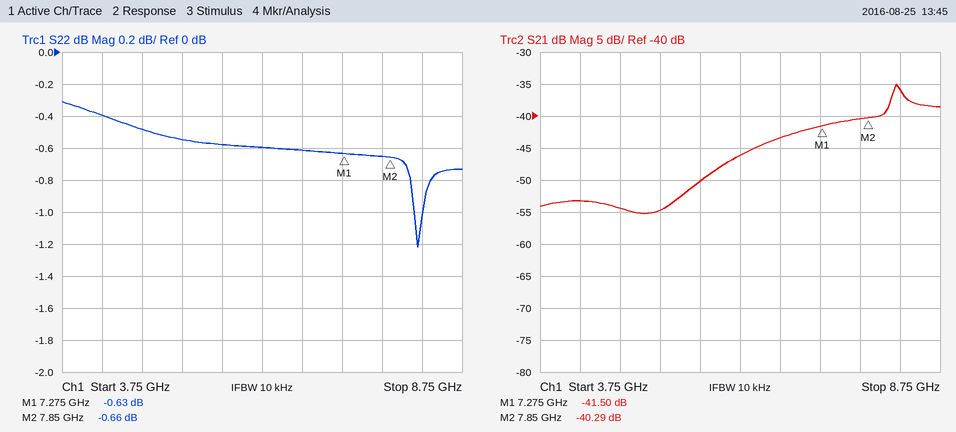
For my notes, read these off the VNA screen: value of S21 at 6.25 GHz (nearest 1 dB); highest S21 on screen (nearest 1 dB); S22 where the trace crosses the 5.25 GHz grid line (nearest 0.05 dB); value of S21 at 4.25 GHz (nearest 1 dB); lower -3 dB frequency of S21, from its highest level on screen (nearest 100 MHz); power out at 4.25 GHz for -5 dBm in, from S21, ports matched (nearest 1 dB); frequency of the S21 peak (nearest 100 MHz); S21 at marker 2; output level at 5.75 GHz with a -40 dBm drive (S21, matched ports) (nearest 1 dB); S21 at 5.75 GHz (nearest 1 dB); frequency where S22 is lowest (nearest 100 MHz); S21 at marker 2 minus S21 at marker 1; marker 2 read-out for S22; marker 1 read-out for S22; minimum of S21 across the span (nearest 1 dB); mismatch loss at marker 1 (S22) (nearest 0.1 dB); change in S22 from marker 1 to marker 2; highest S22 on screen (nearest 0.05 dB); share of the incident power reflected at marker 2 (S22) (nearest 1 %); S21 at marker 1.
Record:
-46 dB
-35 dB
-0.55 dB
-53 dB
8.1 GHz
-58 dBm
8.2 GHz
-40.29 dB
-90 dBm
-50 dB
8.2 GHz
1.21 dB
-0.66 dB
-0.63 dB
-55 dB
8.7 dB
-0.03 dB
-0.30 dB
86 %
-41.50 dB
